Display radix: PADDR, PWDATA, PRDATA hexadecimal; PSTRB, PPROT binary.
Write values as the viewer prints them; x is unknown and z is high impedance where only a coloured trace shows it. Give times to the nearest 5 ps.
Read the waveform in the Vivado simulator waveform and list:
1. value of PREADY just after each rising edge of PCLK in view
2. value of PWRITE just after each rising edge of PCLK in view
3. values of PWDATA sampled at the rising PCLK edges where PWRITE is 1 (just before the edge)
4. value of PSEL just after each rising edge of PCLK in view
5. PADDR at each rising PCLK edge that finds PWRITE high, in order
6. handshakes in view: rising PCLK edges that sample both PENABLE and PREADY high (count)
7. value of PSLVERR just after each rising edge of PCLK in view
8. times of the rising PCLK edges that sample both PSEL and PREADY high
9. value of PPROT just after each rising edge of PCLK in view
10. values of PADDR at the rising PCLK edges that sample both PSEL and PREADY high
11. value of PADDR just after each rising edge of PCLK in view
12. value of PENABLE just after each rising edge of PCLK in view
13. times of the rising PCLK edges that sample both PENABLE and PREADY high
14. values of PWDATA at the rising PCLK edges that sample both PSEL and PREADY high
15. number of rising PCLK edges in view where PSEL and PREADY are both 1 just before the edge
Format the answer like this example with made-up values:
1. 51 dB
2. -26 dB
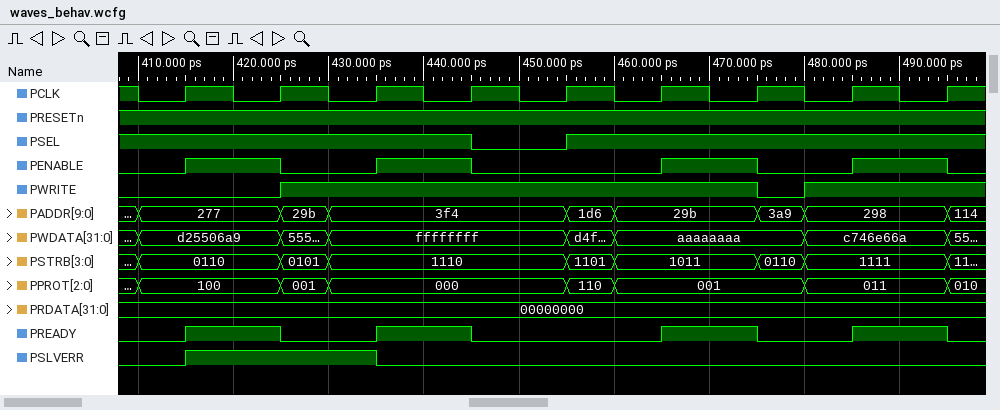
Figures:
1. 1 0 1 0 0 1 0 1 0
2. 0 1 1 1 1 1 0 1 1
3. ffffffff, ffffffff, ffffffff, aaaaaaaa, aaaaaaaa, c746e66a, c746e66a
4. 1 1 1 0 1 1 1 1 1
5. 3f4, 3f4, 3f4, 29b, 29b, 298, 298
6. 4
7. 1 1 0 0 0 0 0 0 0
8. 425 ps, 445 ps, 475 ps, 495 ps
9. 100, 001, 000, 000, 110, 001, 001, 011, 010
10. 277, 3f4, 29b, 298
11. 277, 29b, 3f4, 3f4, 1d6, 29b, 3a9, 298, 114
12. 1 0 1 0 0 1 0 1 0
13. 425 ps, 445 ps, 475 ps, 495 ps
14. d25506a9, ffffffff, aaaaaaaa, c746e66a
15. 4
